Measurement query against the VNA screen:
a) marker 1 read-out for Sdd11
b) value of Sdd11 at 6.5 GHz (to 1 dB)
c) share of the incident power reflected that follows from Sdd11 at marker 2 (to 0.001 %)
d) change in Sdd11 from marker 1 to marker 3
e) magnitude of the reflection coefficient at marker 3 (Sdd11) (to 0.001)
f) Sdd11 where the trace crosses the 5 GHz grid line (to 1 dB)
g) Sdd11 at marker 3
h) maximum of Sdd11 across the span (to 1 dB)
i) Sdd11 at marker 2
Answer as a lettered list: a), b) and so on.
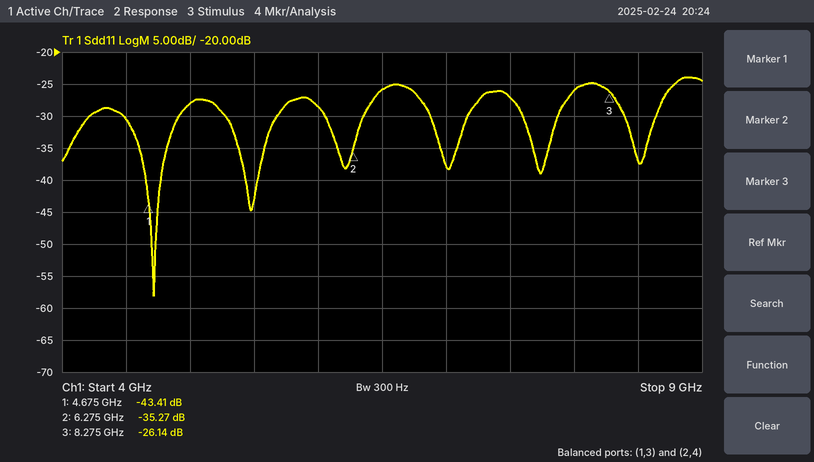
a) -43.41 dB
b) -26 dB
c) 0.030 %
d) 17.27 dB
e) 0.049
f) -28 dB
g) -26.14 dB
h) -24 dB
i) -35.27 dB
